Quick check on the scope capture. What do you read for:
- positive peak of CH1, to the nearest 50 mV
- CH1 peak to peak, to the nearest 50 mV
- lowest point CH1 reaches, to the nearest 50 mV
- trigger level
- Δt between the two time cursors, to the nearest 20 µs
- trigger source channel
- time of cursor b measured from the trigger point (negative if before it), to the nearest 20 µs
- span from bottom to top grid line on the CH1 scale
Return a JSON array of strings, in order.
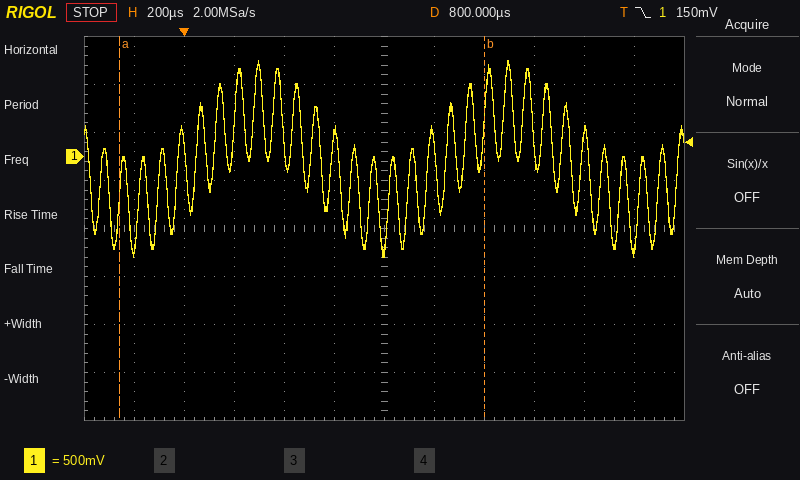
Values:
["1.00 V", "2.05 V", "-1.05 V", "150 mV", "1.46 ms", "CH1", "+1.20 ms", "4 V"]
